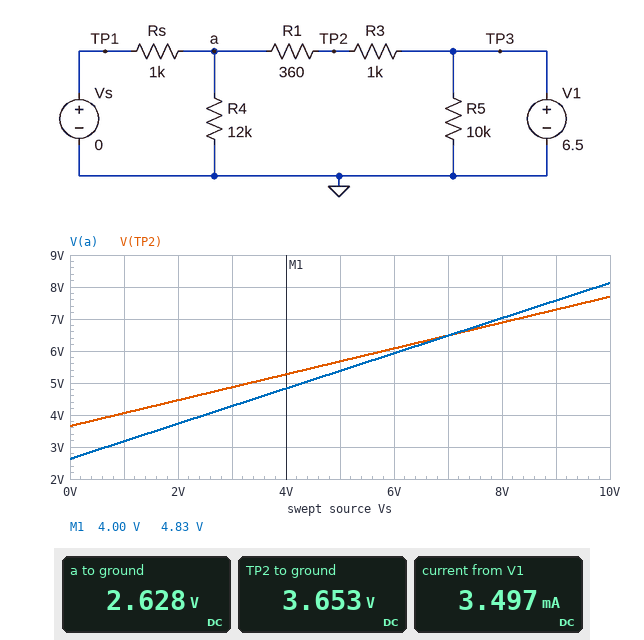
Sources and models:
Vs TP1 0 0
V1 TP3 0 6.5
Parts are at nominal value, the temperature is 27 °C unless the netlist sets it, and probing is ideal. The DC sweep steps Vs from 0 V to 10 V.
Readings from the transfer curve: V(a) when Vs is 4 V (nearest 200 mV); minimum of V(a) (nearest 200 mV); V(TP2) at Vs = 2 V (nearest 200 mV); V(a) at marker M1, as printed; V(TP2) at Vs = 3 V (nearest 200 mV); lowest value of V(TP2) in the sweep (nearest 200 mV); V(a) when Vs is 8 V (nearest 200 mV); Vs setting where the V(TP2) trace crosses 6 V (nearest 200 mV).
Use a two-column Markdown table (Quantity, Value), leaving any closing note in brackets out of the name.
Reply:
| Quantity | Value |
|---|---|
| V(a) when Vs is 4 V | 4.8 V |
| minimum of V(a) | 2.6 V |
| V(TP2) at Vs = 2 V | 4.4 V |
| V(a) at marker M1, as printed | 4.83 V |
| V(TP2) at Vs = 3 V | 4.8 V |
| lowest value of V(TP2) in the sweep | 3.6 V |
| V(a) when Vs is 8 V | 7.0 V |
| Vs setting where the V(TP2) trace crosses 6 V | 5.8 V |
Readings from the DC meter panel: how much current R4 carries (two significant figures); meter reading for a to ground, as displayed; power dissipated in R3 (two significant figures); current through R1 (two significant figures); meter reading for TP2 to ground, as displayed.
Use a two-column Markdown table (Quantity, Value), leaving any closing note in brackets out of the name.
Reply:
| Quantity | Value |
|---|---|
| how much current R4 carries | 220 µA |
| meter reading for a to ground, as displayed | 2.628 V |
| power dissipated in R3 | 8.1 mW |
| current through R1 | 2.8 mA |
| meter reading for TP2 to ground, as displayed | 3.653 V |
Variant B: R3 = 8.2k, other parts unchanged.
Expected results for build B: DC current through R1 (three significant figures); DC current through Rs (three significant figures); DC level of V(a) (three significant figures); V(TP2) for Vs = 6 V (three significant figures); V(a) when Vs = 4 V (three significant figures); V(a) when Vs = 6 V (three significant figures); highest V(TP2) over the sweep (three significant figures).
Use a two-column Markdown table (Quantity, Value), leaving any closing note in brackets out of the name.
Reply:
| Quantity | Value |
|---|---|
| DC current through R1 | 685 µA |
| DC current through Rs | 633 µA |
| DC level of V(a) | 633 mV |
| V(TP2) for Vs = 6 V | 5.67 V |
| V(a) when Vs = 4 V | 3.97 V |
| V(a) when Vs = 6 V | 5.63 V |
| highest V(TP2) over the sweep | 8.86 V |
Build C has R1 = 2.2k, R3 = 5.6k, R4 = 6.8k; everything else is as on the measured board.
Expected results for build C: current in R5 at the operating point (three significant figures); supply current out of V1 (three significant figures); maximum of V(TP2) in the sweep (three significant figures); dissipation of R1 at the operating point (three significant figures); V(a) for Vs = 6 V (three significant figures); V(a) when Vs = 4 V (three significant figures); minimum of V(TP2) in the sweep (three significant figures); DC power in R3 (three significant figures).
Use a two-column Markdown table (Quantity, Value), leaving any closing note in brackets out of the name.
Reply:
| Quantity | Value |
|---|---|
| current in R5 at the operating point | 650 µA |
| supply current out of V1 | 1.40 mA |
| maximum of V(TP2) in the sweep | 7.93 V |
| dissipation of R1 at the operating point | 1.24 mW |
| V(a) for Vs = 6 V | 5.36 V |
| V(a) when Vs = 4 V | 3.79 V |
| minimum of V(TP2) in the sweep | 2.30 V |
| DC power in R3 | 3.15 mW |
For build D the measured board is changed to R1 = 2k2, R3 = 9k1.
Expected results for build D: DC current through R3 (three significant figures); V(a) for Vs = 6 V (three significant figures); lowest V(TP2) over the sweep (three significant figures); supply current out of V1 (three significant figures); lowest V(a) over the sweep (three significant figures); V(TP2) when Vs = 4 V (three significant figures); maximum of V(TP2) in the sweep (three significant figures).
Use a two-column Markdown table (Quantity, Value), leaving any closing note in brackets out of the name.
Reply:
| Quantity | Value |
|---|---|
| DC current through R3 | 532 µA |
| V(a) for Vs = 6 V | 5.61 V |
| lowest V(TP2) over the sweep | 1.66 V |
| supply current out of V1 | 1.18 mA |
| lowest V(a) over the sweep | 491 mV |
| V(TP2) when Vs = 4 V | 4.41 V |
| maximum of V(TP2) in the sweep | 8.53 V |
